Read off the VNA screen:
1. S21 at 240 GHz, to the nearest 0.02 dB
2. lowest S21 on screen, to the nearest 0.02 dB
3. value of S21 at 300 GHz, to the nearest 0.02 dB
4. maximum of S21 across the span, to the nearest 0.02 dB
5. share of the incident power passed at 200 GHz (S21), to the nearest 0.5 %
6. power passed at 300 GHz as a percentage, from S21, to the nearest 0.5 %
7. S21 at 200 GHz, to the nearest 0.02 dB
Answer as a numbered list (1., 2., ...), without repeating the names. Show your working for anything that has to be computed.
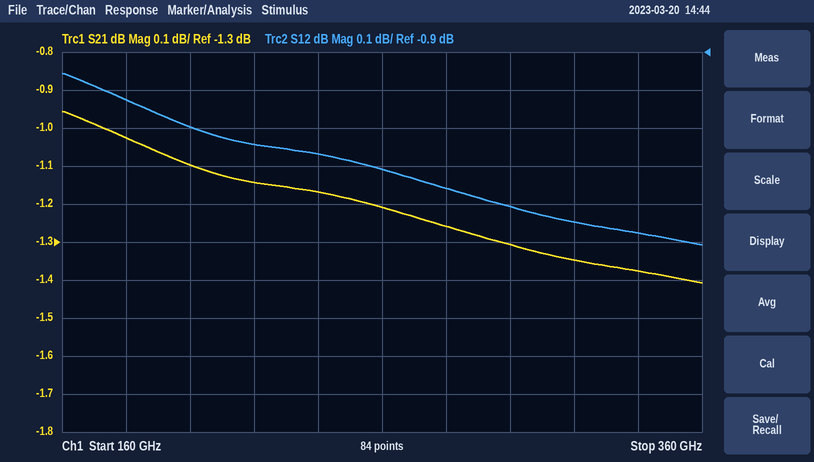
1. -1.16 dB
2. -1.40 dB
3. -1.30 dB
4. -0.96 dB
5. 10^(-1.1/10) ≈ 77.6 %, so 77.5 % to the nearest 0.5 %
6. 10^(-1.3/10) ≈ 74.1 %, so 74.0 % to the nearest 0.5 %
7. -1.10 dB
